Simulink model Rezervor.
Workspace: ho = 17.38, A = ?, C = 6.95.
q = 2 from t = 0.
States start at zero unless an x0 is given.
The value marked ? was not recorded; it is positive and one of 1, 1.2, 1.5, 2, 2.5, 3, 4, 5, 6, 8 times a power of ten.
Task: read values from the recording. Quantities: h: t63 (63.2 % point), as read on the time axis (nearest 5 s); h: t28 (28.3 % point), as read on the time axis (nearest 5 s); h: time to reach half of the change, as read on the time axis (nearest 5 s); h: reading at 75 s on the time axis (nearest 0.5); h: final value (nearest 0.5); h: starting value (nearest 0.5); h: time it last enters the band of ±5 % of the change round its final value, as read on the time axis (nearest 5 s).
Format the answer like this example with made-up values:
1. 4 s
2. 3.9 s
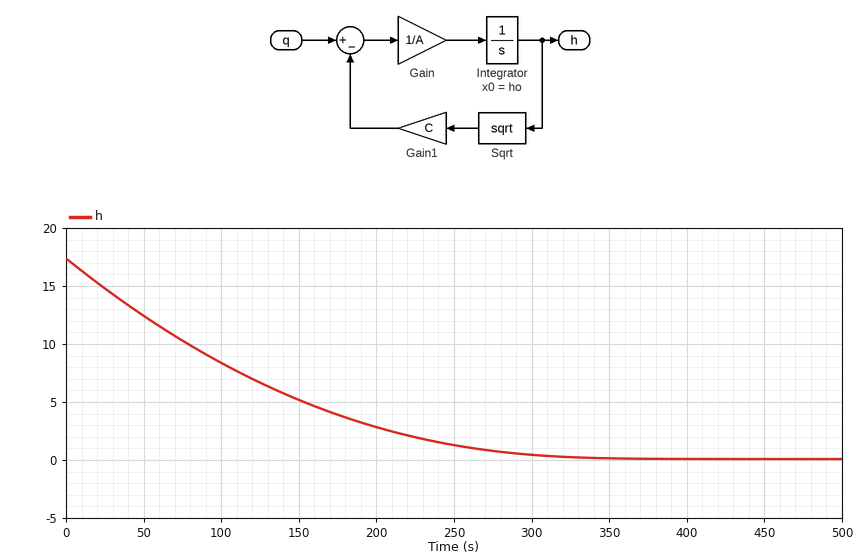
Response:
1. 130 s
2. 50 s
3. 95 s
4. 10.5
5. 0.0
6. 17.5
7. 265 s
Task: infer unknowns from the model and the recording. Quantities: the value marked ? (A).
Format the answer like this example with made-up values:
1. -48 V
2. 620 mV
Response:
1. 250
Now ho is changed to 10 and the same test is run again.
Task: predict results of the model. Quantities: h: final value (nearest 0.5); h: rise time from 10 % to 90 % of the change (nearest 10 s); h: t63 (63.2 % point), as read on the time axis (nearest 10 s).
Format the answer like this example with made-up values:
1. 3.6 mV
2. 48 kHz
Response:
1. 0.0
2. 170 s
3. 100 s
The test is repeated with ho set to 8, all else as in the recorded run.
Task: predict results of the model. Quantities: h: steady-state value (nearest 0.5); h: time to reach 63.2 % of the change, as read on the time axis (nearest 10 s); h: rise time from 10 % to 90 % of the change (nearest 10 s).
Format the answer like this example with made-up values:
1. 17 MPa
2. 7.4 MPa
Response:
1. 0.0
2. 90 s
3. 150 s
